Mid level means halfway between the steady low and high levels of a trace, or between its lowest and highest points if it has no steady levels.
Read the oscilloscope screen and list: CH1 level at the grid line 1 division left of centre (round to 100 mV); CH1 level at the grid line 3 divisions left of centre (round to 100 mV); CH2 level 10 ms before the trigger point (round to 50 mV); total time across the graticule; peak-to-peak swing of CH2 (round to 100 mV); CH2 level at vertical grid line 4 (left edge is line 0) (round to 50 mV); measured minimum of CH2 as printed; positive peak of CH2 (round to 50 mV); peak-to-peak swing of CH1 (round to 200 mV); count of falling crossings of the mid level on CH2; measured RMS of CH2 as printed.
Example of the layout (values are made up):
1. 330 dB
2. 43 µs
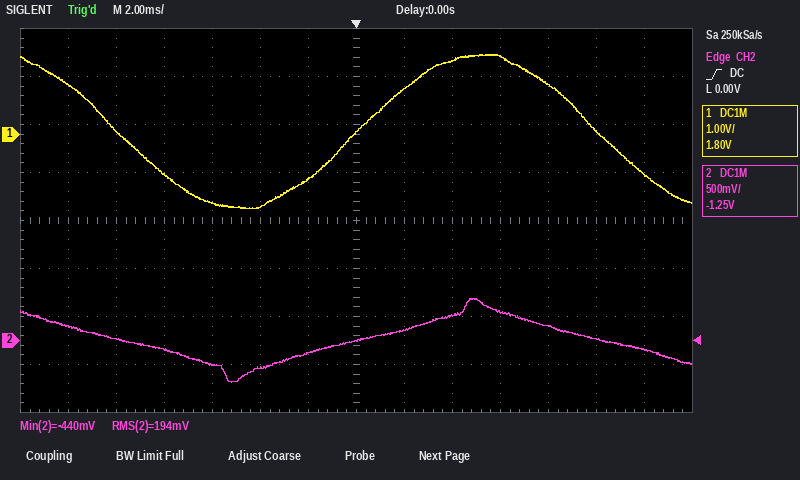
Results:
1. -900 mV
2. -1.4 V
3. 0 mV
4. 28 ms
5. 900 mV
6. -250 mV
7. -440 mV
8. 450 mV
9. 3.2 V
10. 2
11. 194 mV
